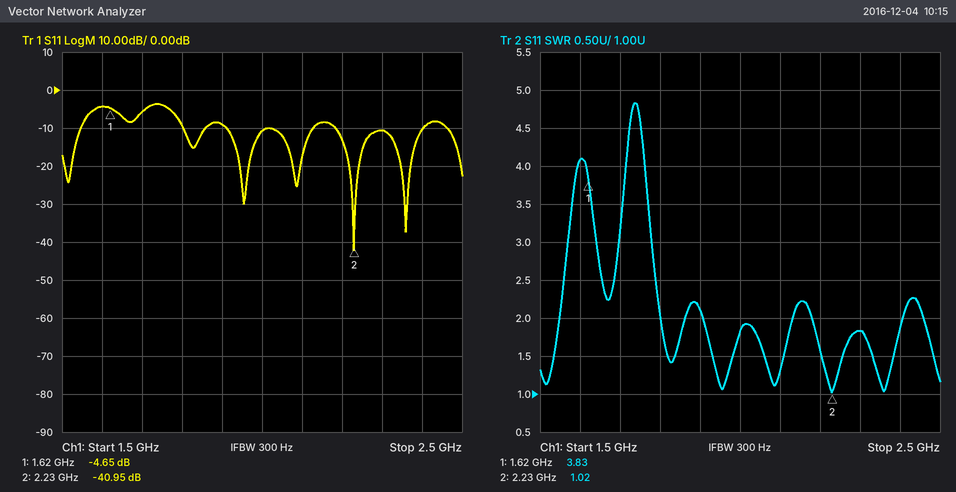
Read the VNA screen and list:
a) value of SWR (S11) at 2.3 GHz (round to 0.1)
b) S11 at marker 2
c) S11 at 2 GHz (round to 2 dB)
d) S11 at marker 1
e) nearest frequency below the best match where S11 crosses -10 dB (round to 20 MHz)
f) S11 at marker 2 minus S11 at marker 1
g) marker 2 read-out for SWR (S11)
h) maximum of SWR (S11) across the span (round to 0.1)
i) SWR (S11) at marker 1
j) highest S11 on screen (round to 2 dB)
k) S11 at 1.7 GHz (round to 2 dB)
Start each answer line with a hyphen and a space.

- 1.8
- -40.95 dB
- -10 dB
- -4.65 dB
- 2.18 GHz
- -36.30 dB
- 1.02
- 4.8
- 3.83
- -4 dB
- -6 dB
